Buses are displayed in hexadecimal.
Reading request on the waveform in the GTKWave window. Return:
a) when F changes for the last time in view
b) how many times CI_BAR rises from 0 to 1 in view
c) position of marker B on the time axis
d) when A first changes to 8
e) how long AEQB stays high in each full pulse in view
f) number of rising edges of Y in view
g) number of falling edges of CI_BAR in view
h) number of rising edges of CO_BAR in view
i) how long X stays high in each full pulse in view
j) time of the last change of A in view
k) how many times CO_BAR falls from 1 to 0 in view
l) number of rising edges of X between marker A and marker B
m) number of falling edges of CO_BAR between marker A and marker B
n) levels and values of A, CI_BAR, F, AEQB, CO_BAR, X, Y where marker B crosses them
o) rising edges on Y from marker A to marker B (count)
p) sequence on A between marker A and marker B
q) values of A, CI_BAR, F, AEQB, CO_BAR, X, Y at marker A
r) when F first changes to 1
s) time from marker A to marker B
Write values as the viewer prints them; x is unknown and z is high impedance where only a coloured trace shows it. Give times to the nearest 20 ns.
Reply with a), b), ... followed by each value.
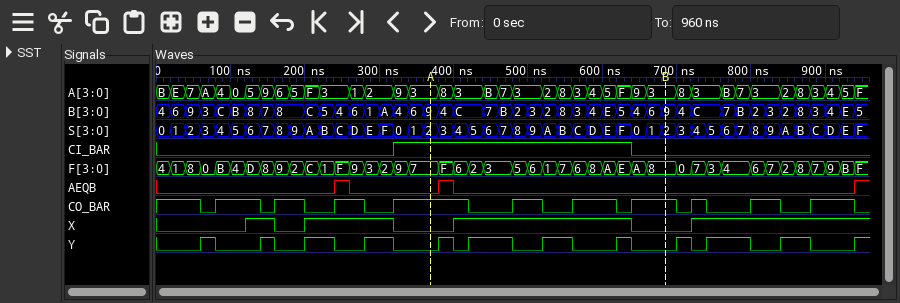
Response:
a) 940 ns
b) 1
c) 680 ns
d) 380 ns
e) 20 ns, 20 ns
f) 12
g) 1
h) 10
i) 40 ns, 120 ns, 240 ns
j) 940 ns
k) 11
l) 1
m) 3
n) A=3, CI_BAR=0, F=8, AEQB=0, CO_BAR=1, X=0, Y=0
o) 4
p) 3, 8, 3, B, 7, 3, 2, 8, 3, 4, 5, F, 9, 3
q) A=3, CI_BAR=1, F=7, AEQB=0, CO_BAR=1, X=0, Y=0
r) 20 ns
s) 320 ns
